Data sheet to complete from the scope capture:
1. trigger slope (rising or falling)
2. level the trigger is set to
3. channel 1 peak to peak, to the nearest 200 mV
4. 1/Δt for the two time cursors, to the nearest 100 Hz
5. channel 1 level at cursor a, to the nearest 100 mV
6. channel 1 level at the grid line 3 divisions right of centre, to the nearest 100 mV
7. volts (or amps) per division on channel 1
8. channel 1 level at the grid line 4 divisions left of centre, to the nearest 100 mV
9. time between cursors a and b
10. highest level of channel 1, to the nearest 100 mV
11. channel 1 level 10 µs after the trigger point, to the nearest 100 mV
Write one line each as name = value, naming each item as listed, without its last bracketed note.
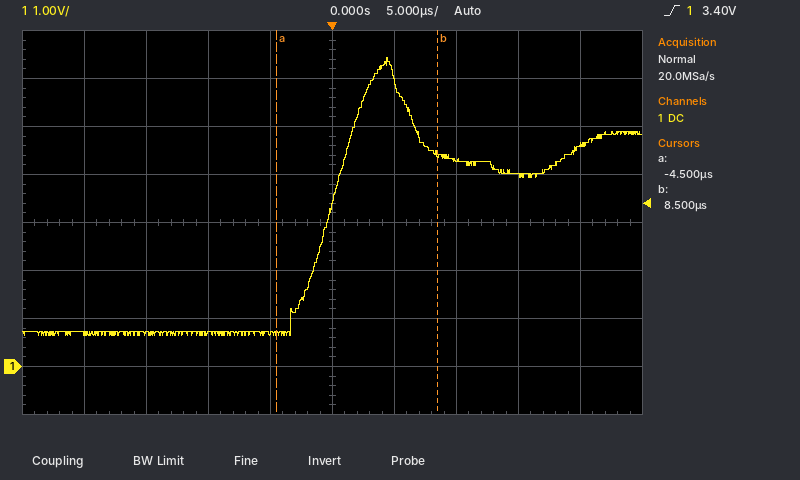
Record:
trigger slope = rising
level the trigger is set to = 3.40 V
channel 1 peak to peak, to the nearest 200 mV = 5.8 V
1/Δt for the two time cursors, to the nearest 100 Hz = 76.9 kHz
channel 1 level at cursor a, to the nearest 100 mV = 700 mV
channel 1 level at the grid line 3 divisions right of centre, to the nearest 100 mV = 4.0 V
volts (or amps) per division on channel 1 = 1 V
channel 1 level at the grid line 4 divisions left of centre, to the nearest 100 mV = 700 mV
time between cursors a and b = 13.0 µs
highest level of channel 1, to the nearest 100 mV = 6.4 V
channel 1 level 10 µs after the trigger point, to the nearest 100 mV = 4.3 V
